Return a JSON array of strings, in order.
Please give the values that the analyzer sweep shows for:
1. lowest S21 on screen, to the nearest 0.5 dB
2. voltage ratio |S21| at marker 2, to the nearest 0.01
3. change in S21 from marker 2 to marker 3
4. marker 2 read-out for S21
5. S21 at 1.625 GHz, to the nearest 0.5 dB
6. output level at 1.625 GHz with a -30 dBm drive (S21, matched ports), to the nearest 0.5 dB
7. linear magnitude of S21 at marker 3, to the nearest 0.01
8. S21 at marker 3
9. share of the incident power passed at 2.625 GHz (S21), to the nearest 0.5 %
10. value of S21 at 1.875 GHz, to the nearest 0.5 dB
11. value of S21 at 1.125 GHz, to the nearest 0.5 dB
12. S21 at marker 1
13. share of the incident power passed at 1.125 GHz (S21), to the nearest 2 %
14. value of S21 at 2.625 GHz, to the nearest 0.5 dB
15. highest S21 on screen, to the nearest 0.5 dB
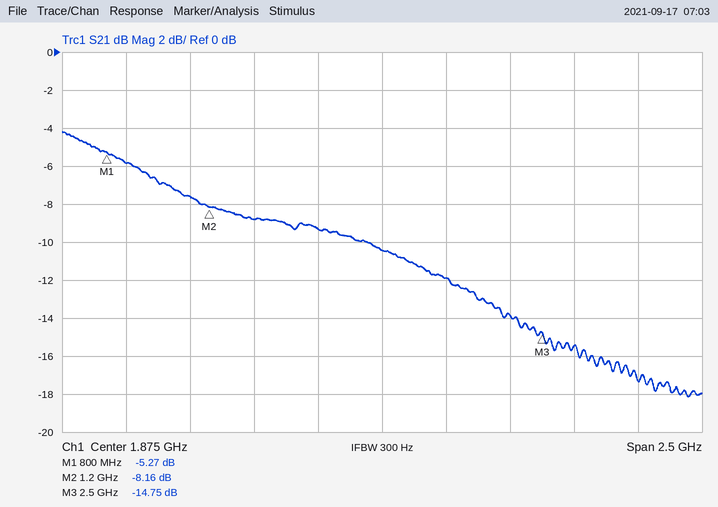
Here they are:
["-18.0 dB", "0.39", "-6.59 dB", "-8.16 dB", "-9.5 dB", "-39.5 dBm", "0.18", "-14.75 dB", "3.0 %", "-10.5 dB", "-7.5 dB", "-5.27 dB", "18 %", "-15.5 dB", "-4.0 dB"]
